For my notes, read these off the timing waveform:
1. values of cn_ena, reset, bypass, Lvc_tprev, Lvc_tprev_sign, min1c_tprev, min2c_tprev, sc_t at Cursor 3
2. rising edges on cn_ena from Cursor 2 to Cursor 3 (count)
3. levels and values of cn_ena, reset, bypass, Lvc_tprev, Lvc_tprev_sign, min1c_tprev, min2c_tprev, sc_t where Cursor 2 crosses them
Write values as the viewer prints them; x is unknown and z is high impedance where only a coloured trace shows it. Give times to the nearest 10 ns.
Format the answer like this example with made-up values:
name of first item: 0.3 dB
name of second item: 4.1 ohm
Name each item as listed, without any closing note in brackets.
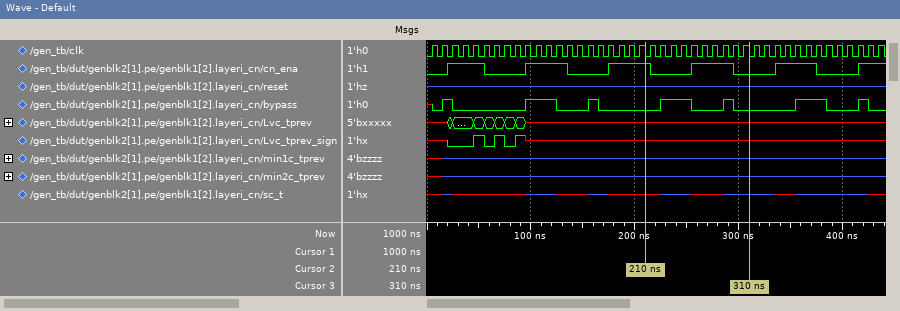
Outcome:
values of cn_ena, reset, bypass, Lvc_tprev, Lvc_tprev_sign, min1c_tprev, min2c_tprev, sc_t at Cursor 3: cn_ena=0, reset=z, bypass=0, Lvc_tprev=x, Lvc_tprev_sign=x, min1c_tprev=z, min2c_tprev=z, sc_t=z
rising edges on cn_ena from Cursor 2 to Cursor 3: 1
levels and values of cn_ena, reset, bypass, Lvc_tprev, Lvc_tprev_sign, min1c_tprev, min2c_tprev, sc_t where Cursor 2 crosses them: cn_ena=1, reset=z, bypass=0, Lvc_tprev=x, Lvc_tprev_sign=x, min1c_tprev=z, min2c_tprev=z, sc_t=x
